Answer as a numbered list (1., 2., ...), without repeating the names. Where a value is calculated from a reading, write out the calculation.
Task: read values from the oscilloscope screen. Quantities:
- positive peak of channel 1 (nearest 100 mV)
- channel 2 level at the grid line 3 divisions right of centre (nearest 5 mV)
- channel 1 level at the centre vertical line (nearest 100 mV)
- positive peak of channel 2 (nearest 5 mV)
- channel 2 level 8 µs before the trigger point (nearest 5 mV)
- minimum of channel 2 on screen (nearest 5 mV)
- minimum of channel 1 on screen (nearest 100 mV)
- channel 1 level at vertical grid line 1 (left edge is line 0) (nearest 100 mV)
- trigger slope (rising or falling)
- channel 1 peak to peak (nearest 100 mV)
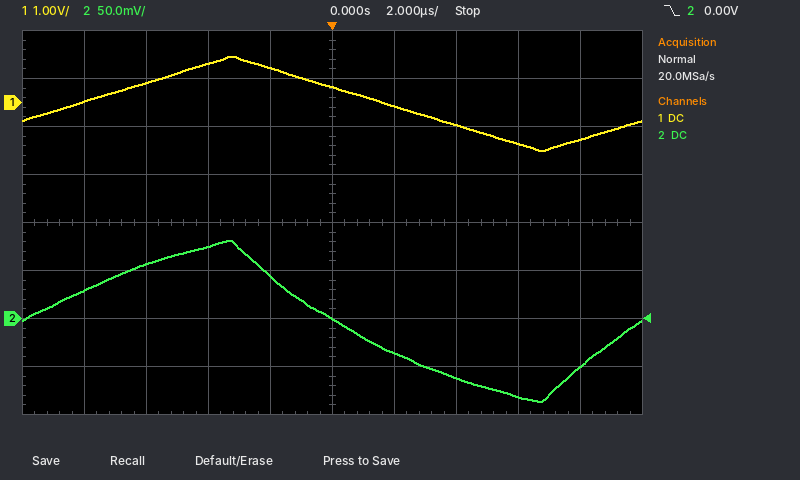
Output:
1. 1.0 V
2. -80 mV
3. 300 mV
4. 80 mV
5. 30 mV
6. -85 mV
7. -1.0 V
8. 0.0 V
9. falling
10. 1.0 V − (-1.0 V) = 2.0 V
